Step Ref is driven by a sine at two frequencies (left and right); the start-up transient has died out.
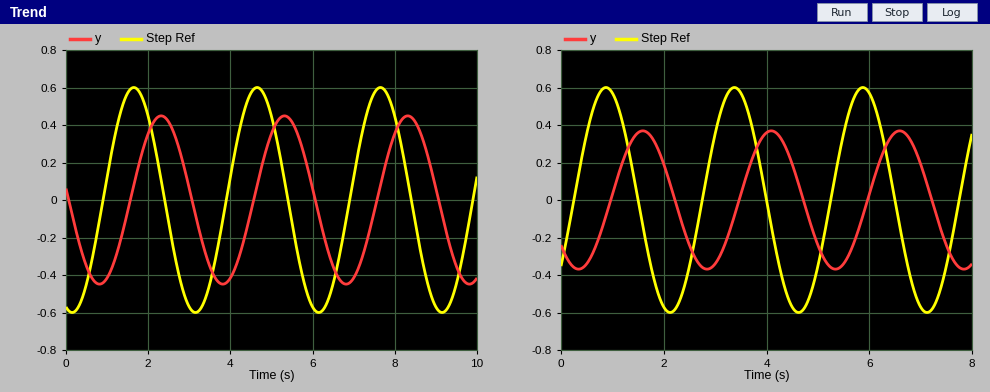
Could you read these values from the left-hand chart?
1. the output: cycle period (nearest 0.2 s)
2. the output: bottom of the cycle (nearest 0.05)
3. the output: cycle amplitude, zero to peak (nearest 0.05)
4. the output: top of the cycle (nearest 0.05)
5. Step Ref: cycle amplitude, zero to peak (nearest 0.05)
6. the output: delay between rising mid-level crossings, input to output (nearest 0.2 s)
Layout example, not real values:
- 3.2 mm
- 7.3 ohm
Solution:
- 3.0 s
- -0.45
- 0.45
- 0.45
- 0.60
- 0.6 s
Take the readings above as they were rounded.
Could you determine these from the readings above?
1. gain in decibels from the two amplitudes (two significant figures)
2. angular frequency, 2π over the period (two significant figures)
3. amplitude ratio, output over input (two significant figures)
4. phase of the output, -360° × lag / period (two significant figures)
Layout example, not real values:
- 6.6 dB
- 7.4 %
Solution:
- -2.5 dB
- 2.1 rad/s
- 0.75
- -72°
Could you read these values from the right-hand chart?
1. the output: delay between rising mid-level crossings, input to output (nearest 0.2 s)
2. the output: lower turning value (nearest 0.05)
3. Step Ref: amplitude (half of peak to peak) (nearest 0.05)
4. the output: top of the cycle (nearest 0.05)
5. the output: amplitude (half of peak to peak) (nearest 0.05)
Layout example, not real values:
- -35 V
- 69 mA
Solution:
- 0.8 s
- -0.35
- 0.60
- 0.35
- 0.35
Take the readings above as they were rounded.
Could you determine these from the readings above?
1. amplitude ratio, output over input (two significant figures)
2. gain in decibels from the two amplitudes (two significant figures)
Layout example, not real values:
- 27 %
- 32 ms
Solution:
- 0.58
- -4.7 dB
